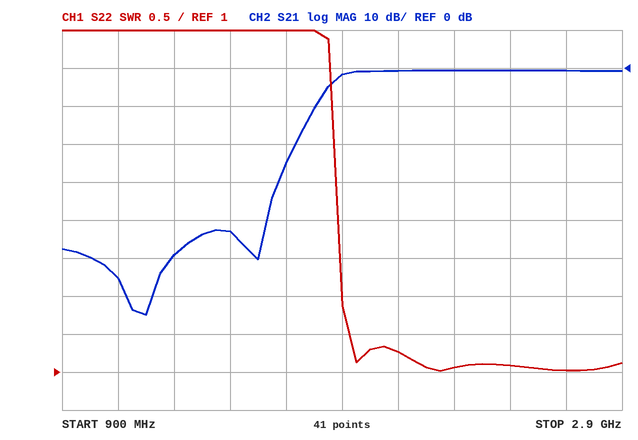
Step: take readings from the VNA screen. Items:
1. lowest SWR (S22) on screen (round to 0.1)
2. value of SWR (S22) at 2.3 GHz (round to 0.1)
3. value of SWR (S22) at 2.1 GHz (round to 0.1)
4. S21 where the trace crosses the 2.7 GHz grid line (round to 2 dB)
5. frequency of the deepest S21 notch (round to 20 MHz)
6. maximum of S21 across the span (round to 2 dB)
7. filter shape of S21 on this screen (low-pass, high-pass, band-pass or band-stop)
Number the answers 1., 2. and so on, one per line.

1. 1.0
2. 1.1
3. 1.3
4. 0 dB
5. 1.20 GHz
6. 0 dB
7. high-pass
